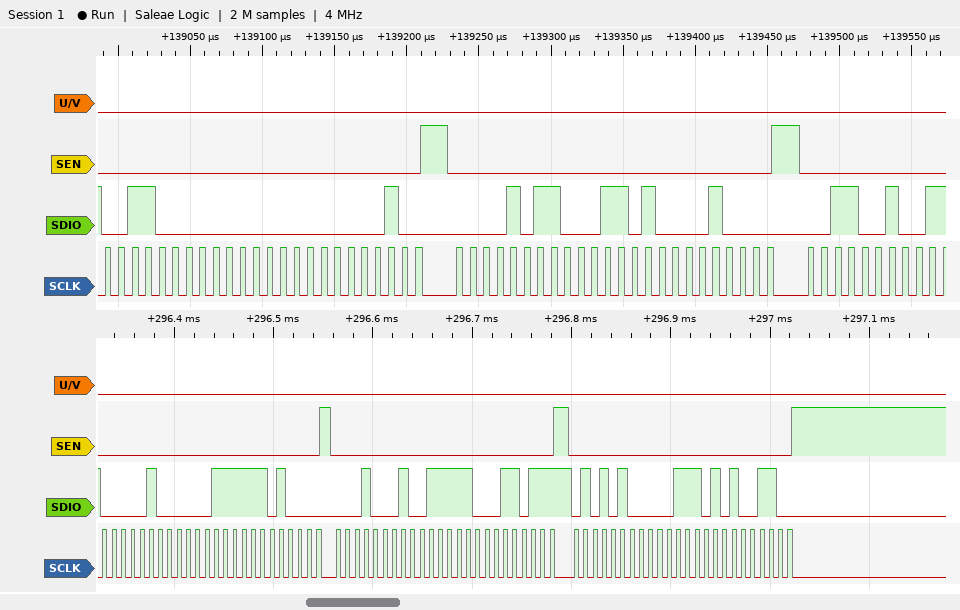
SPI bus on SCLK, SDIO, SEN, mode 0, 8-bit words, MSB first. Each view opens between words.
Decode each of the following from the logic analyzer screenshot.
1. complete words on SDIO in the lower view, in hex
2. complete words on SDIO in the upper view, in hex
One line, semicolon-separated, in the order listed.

04, 0F, D0, 11, 3E, 37, 54, 1D, 4C; 30, 00, 04, 0B, 1A, 10, 32
